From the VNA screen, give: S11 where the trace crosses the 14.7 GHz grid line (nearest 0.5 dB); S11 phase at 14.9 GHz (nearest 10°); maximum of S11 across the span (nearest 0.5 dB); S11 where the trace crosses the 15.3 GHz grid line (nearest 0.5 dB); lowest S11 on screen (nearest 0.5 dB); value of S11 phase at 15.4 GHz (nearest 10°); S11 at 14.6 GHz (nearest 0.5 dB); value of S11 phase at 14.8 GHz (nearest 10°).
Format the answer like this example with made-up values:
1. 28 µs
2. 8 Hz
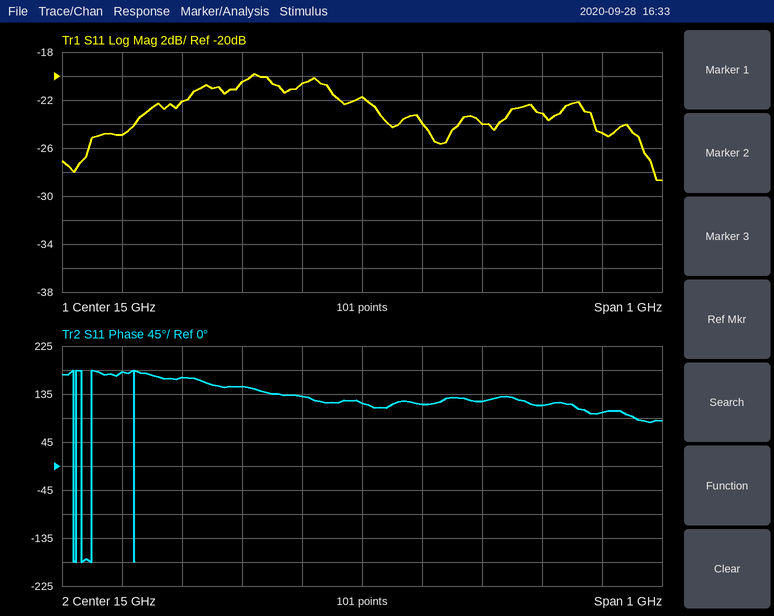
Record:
1. -22.0 dB
2. 130°
3. -20.0 dB
4. -23.0 dB
5. -28.5 dB
6. 100°
7. -25.0 dB
8. 150°
